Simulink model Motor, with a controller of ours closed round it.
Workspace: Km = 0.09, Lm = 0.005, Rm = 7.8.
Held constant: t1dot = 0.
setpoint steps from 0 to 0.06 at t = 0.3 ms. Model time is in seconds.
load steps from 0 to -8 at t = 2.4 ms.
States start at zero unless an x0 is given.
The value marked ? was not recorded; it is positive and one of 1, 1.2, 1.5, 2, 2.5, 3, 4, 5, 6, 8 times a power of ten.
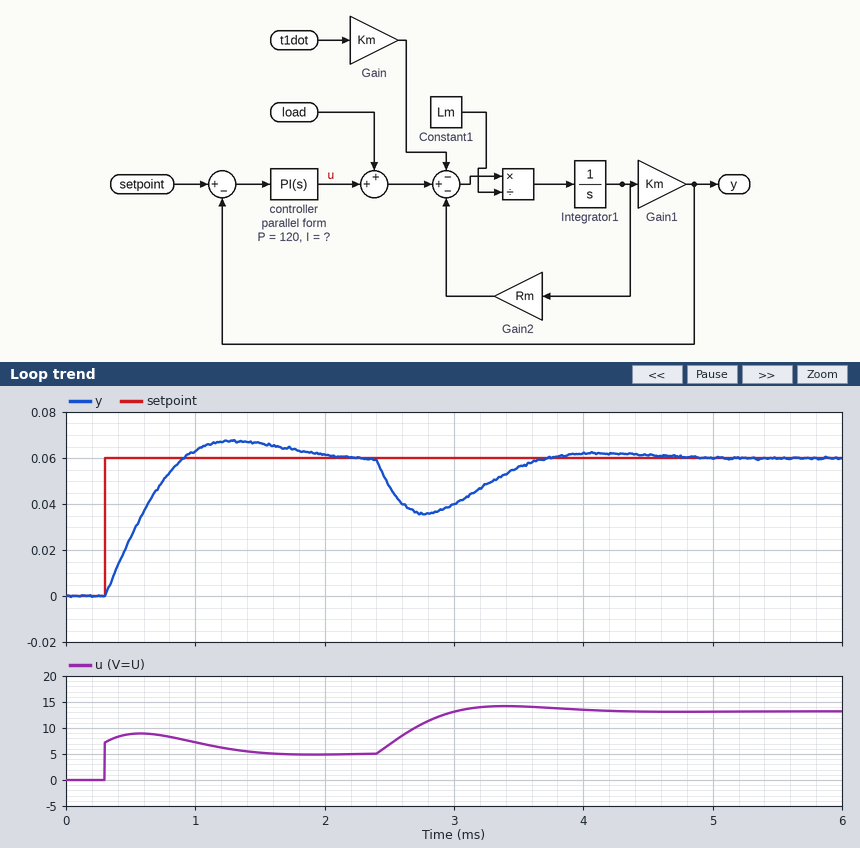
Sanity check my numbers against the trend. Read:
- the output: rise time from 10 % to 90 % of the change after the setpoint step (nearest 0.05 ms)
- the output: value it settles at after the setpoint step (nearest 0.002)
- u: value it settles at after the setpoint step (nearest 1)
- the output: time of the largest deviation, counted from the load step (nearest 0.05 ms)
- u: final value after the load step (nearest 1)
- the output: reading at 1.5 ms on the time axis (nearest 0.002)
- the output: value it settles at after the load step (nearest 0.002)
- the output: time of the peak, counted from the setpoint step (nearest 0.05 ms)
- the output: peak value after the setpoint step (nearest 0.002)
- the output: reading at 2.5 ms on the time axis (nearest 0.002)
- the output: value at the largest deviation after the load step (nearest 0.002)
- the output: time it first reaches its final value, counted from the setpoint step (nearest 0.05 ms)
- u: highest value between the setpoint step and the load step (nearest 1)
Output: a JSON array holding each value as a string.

["0.45 ms", "0.060", "5", "0.40 ms", "13", "0.066", "0.060", "1.00 ms", "0.068", "0.048", "0.036", "0.60 ms", "9"]
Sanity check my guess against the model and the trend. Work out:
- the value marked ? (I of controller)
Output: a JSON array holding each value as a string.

["500000"]
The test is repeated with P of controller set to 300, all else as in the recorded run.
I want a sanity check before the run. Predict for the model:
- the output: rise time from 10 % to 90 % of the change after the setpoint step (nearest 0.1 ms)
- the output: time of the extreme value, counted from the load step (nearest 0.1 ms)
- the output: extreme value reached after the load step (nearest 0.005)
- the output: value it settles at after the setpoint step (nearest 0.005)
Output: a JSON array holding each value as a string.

["0.4 ms", "0.3 ms", "0.045", "0.060"]
